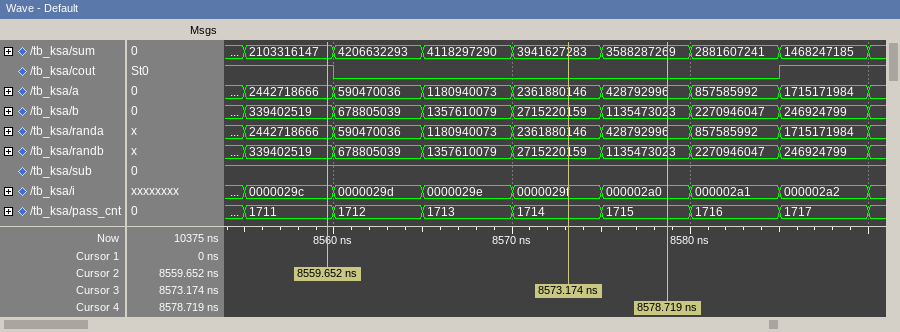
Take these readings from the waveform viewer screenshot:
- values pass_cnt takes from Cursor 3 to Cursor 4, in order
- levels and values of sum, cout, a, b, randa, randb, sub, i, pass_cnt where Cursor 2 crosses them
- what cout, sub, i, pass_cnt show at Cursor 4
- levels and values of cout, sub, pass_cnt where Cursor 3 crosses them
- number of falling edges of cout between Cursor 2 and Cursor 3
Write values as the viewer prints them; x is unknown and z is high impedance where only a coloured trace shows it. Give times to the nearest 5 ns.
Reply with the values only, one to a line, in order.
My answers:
1714, 1715
sum=2103316147, cout=1, a=2442718666, b=339402519, randa=2442718666, randb=339402519, sub=1, i=0000029c, pass_cnt=1711
cout=0, sub=1, i=000002a0, pass_cnt=1715
cout=0, sub=1, pass_cnt=1714
1
